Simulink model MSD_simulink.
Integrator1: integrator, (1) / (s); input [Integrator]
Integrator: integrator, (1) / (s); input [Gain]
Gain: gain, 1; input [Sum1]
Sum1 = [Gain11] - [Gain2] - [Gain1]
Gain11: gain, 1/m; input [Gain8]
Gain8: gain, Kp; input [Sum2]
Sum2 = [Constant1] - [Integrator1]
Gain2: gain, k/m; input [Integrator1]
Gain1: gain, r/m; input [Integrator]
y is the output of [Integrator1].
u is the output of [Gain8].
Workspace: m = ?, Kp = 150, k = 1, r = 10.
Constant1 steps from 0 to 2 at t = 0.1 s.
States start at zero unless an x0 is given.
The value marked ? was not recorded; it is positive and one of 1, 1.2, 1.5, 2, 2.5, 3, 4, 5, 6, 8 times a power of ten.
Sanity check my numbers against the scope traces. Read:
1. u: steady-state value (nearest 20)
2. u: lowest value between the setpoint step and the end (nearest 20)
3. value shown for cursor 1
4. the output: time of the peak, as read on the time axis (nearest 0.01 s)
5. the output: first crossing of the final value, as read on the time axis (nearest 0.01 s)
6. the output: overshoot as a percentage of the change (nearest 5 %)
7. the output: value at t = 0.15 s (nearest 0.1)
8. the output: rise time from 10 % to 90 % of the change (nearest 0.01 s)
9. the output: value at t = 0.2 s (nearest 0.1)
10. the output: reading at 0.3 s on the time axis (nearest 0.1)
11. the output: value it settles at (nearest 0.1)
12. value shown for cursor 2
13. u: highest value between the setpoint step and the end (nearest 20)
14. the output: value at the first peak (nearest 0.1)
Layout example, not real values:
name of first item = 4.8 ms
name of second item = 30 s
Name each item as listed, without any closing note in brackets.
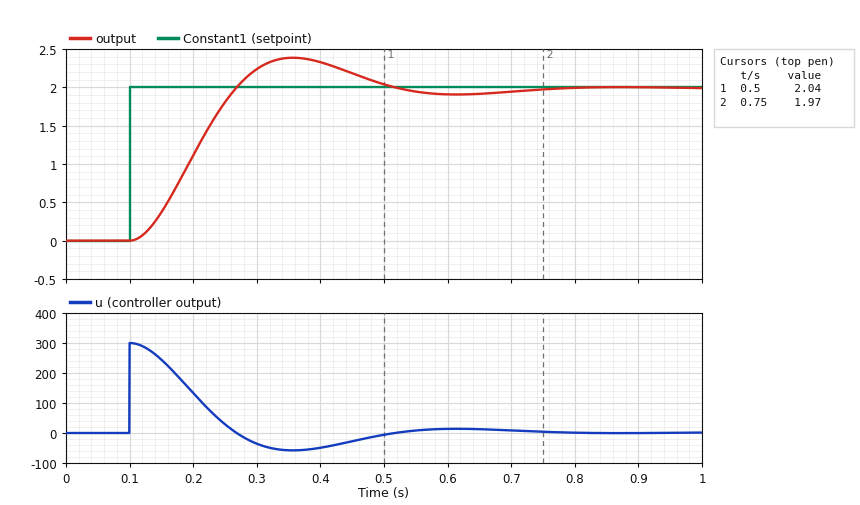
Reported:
u: steady-state value = 0
u: lowest value between the setpoint step and the end = -60
value shown for cursor 1 = 2.04
the output: time of the peak, as read on the time axis = 0.36 s
the output: first crossing of the final value, as read on the time axis = 0.27 s
the output: overshoot as a percentage of the change = 20 %
the output: value at t = 0.15 s = 0.4
the output: rise time from 10 % to 90 % of the change = 0.11 s
the output: value at t = 0.2 s = 1.1
the output: reading at 0.3 s on the time axis = 2.2
the output: value it settles at = 2.0
value shown for cursor 2 = 1.97
u: highest value between the setpoint step and the end = 300
the output: value at the first peak = 2.4
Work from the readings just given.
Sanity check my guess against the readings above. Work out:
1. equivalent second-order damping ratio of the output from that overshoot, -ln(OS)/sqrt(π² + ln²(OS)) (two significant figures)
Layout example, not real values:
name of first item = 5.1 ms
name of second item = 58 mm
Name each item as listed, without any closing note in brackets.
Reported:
equivalent second-order damping ratio of the output from that overshoot, -ln(OS)/sqrt(π² + ln²(OS)) = 0.46
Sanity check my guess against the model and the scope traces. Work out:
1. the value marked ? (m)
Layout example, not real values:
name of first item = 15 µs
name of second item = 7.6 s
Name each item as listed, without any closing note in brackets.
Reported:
the value marked ? = 0.8
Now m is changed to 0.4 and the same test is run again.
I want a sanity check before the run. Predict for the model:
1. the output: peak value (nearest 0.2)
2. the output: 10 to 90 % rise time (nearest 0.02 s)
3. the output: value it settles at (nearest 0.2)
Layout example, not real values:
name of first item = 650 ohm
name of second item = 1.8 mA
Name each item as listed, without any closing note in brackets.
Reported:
the output: peak value = 2.2
the output: 10 to 90 % rise time = 0.10 s
the output: value it settles at = 2.0
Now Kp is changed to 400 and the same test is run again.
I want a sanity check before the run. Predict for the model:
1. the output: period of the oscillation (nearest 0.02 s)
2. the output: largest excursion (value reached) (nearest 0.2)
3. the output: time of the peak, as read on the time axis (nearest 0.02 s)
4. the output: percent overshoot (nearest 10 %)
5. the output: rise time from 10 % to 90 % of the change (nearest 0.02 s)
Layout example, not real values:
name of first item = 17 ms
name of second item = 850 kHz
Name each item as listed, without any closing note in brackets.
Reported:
the output: period of the oscillation = 0.30 s
the output: largest excursion (value reached) = 2.8
the output: time of the peak, as read on the time axis = 0.24 s
the output: percent overshoot = 40 %
the output: rise time from 10 % to 90 % of the change = 0.06 s
